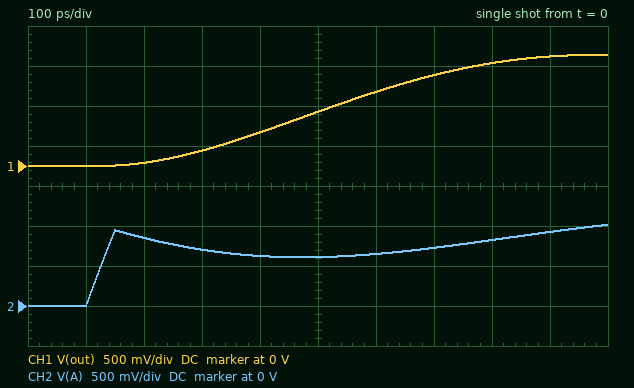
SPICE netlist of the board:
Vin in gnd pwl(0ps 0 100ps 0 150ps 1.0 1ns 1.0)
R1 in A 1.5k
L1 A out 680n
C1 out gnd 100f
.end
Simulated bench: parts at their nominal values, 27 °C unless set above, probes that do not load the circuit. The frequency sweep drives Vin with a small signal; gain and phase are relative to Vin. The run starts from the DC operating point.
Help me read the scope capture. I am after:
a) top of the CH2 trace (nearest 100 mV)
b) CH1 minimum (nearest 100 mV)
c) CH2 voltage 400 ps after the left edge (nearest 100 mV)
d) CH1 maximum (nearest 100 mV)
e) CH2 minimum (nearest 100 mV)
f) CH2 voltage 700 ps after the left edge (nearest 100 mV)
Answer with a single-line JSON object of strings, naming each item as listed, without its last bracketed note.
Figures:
{"top of the CH2 trace": "1.0 V", "CH1 minimum": "0 V", "CH2 voltage 400 ps after the left edge": "600 mV", "CH1 maximum": "1.4 V", "CH2 minimum": "0 V", "CH2 voltage 700 ps after the left edge": "700 mV"}
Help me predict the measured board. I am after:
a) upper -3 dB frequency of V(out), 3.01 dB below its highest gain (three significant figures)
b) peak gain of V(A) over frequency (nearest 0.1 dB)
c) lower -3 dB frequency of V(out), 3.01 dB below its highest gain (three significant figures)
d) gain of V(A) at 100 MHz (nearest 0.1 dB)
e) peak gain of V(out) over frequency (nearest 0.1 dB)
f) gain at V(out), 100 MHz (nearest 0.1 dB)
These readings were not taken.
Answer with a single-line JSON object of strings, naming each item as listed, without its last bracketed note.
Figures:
{"upper -3 dB frequency of V(out), 3.01 dB below its highest gain": "718 MHz", "peak gain of V(A) over frequency": "0 dB", "lower -3 dB frequency of V(out), 3.01 dB below its highest gain": "325 MHz", "gain of V(A) at 100 MHz": "0 dB", "peak gain of V(out) over frequency": "5.2 dB", "gain at V(out), 100 MHz": "0.2 dB"}
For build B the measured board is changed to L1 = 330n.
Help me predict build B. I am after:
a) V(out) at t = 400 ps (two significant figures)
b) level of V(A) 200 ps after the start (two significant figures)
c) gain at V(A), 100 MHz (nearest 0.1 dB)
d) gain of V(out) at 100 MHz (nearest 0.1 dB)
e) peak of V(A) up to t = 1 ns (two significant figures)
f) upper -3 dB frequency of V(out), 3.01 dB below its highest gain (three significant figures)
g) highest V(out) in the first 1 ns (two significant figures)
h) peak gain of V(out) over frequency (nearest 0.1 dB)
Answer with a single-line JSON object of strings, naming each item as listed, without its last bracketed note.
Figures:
{"V(out) at t = 400 ps": "660 mV", "level of V(A) 200 ps after the start": "720 mV", "gain at V(A), 100 MHz": "0 dB", "gain of V(out) at 100 MHz": "0.1 dB", "peak of V(A) up to t = 1 ns": "1.1 V", "upper -3 dB frequency of V(out), 3.01 dB below its highest gain": "1.04 GHz", "highest V(out) in the first 1 ns": "1.2 V", "peak gain of V(out) over frequency": "2.5 dB"}
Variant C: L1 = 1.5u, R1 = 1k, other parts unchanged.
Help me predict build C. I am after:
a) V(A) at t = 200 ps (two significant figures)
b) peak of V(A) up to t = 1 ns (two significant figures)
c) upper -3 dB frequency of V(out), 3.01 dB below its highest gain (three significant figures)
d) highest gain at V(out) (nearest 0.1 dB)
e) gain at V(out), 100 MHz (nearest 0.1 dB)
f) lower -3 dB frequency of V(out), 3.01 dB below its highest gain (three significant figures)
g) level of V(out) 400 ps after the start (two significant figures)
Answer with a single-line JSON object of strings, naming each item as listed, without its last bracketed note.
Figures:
{"V(A) at t = 200 ps": "950 mV", "peak of V(A) up to t = 1 ns": "980 mV", "upper -3 dB frequency of V(out), 3.01 dB below its highest gain": "454 MHz", "highest gain at V(out)": "11.8 dB", "gain at V(out), 100 MHz": "0.5 dB", "lower -3 dB frequency of V(out), 3.01 dB below its highest gain": "346 MHz", "level of V(out) 400 ps after the start": "230 mV"}
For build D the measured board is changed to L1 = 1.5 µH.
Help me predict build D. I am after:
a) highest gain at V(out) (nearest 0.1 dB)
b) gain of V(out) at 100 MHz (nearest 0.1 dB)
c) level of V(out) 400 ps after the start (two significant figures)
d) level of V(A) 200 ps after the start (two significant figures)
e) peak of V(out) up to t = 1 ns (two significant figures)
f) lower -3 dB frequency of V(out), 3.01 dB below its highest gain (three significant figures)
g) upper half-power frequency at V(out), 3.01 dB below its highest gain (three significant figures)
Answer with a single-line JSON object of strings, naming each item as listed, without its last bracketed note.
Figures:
{"highest gain at V(out)": "8.4 dB", "gain of V(out) at 100 MHz": "0.5 dB", "level of V(out) 400 ps after the start": "220 mV", "level of V(A) 200 ps after the start": "930 mV", "peak of V(out) up to t = 1 ns": "1.3 V", "lower -3 dB frequency of V(out), 3.01 dB below its highest gain": "303 MHz", "upper half-power frequency at V(out), 3.01 dB below its highest gain": "469 MHz"}
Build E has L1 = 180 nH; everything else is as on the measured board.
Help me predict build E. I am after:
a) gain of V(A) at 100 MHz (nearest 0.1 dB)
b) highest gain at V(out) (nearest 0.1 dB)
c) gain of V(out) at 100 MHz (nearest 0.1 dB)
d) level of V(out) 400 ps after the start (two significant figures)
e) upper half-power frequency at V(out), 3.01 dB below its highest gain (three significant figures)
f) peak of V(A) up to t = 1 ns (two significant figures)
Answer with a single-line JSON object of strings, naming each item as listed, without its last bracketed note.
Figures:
{"gain of V(A) at 100 MHz": "0 dB", "highest gain at V(out)": "0.7 dB", "gain of V(out) at 100 MHz": "0 dB", "level of V(out) 400 ps after the start": "830 mV", "upper half-power frequency at V(out), 3.01 dB below its highest gain": "1.35 GHz", "peak of V(A) up to t = 1 ns": "1.1 V"}
